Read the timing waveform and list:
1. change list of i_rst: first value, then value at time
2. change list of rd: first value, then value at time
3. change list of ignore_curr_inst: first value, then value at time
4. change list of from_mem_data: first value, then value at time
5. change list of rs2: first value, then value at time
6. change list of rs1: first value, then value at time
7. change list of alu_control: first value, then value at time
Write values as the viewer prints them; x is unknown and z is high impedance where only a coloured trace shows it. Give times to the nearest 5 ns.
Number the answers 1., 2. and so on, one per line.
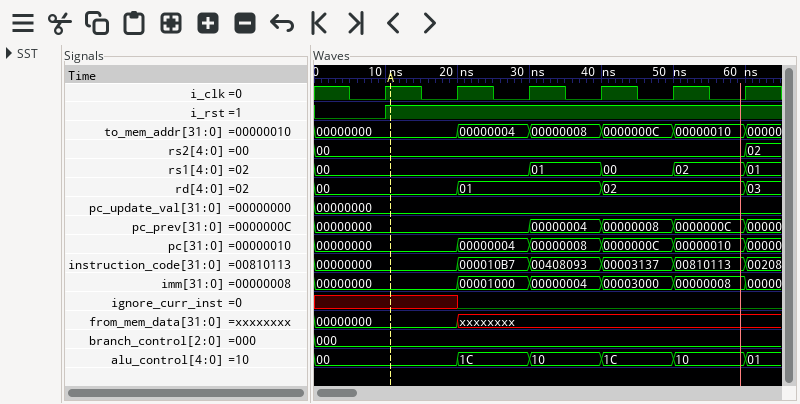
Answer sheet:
1. 0, 1 at 10 ns
2. 00, 01 at 20 ns, 02 at 40 ns, 03 at 60 ns
3. x, 0 at 20 ns
4. 00000000, xxxxxxxx at 20 ns
5. 00, 02 at 60 ns
6. 00, 01 at 30 ns, 00 at 40 ns, 02 at 50 ns, 01 at 60 ns
7. 00, 1C at 20 ns, 10 at 30 ns, 1C at 40 ns, 10 at 50 ns, 01 at 60 ns
